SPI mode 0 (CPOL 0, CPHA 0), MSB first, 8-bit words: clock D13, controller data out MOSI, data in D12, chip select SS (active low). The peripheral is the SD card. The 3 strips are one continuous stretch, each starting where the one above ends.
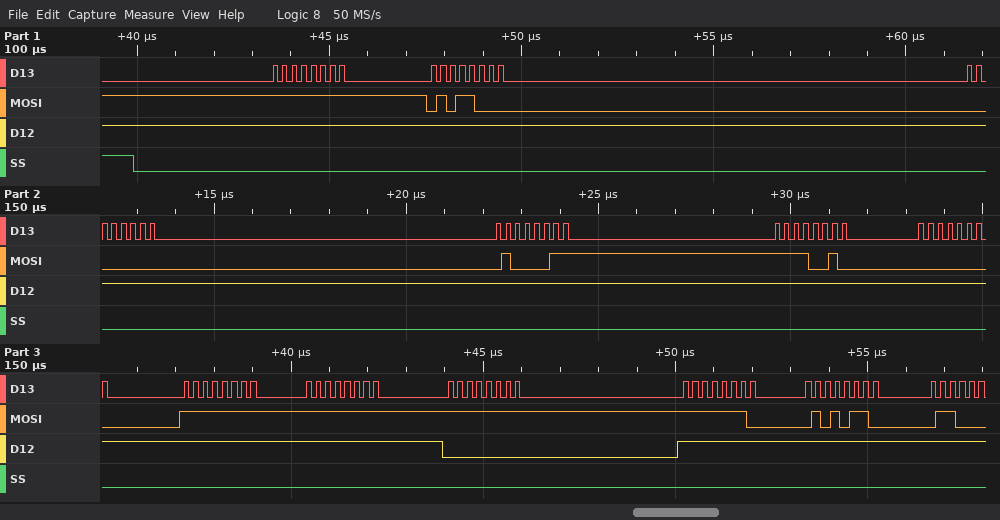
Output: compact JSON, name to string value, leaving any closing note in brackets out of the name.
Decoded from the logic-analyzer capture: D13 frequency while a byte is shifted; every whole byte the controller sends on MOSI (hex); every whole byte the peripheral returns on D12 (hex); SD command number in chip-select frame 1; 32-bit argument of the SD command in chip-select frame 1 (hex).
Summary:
{"D13 frequency while a byte is shifted": "4 MHz", "every whole byte the controller sends on MOSI": "FF 58 00 43 F2 00 FF FF FF FE 56", "every whole byte the peripheral returns on D12": "FF FF FF FF FF FF FF FF 00 FF FF", "SD command number in chip-select frame 1": "CMD24", "32-bit argument of the SD command in chip-select frame 1": "0x0043F200"}
